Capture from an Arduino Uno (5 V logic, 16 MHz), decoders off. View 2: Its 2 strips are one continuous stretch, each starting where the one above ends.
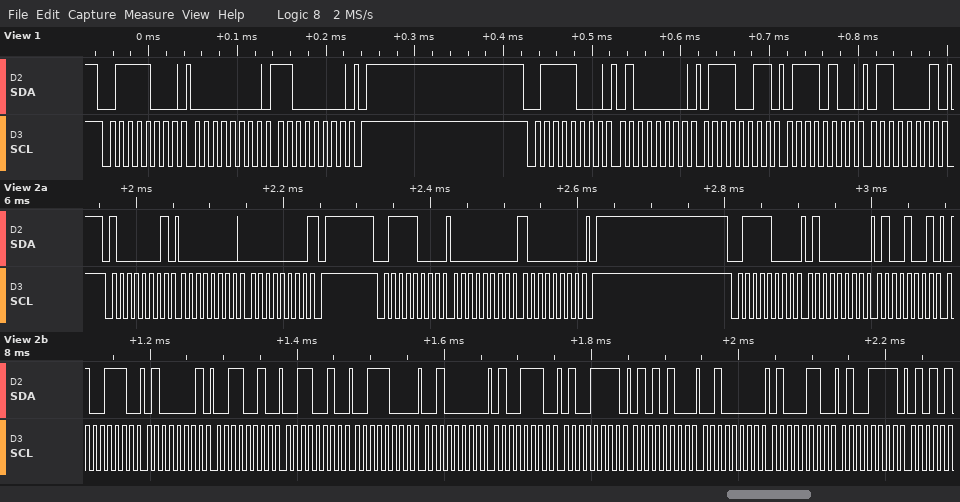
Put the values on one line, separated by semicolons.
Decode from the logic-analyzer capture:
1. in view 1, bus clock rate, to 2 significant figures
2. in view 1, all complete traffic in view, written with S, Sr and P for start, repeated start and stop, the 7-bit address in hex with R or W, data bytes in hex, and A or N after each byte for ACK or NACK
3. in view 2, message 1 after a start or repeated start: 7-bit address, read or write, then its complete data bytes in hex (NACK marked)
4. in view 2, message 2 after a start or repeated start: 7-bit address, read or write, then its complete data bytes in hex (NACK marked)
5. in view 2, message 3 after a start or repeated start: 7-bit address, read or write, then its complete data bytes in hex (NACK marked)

100 kHz; S 3CW A 00 A C0 A P S 3CW A 40 A 73 A 74 A 61 A; 0x40 read: 00 00 NACK; 0x3C write: 00 80; 0x3C write: 40 49 4E 41 32 32 38 20 4E 4F 54 20 46 4F
